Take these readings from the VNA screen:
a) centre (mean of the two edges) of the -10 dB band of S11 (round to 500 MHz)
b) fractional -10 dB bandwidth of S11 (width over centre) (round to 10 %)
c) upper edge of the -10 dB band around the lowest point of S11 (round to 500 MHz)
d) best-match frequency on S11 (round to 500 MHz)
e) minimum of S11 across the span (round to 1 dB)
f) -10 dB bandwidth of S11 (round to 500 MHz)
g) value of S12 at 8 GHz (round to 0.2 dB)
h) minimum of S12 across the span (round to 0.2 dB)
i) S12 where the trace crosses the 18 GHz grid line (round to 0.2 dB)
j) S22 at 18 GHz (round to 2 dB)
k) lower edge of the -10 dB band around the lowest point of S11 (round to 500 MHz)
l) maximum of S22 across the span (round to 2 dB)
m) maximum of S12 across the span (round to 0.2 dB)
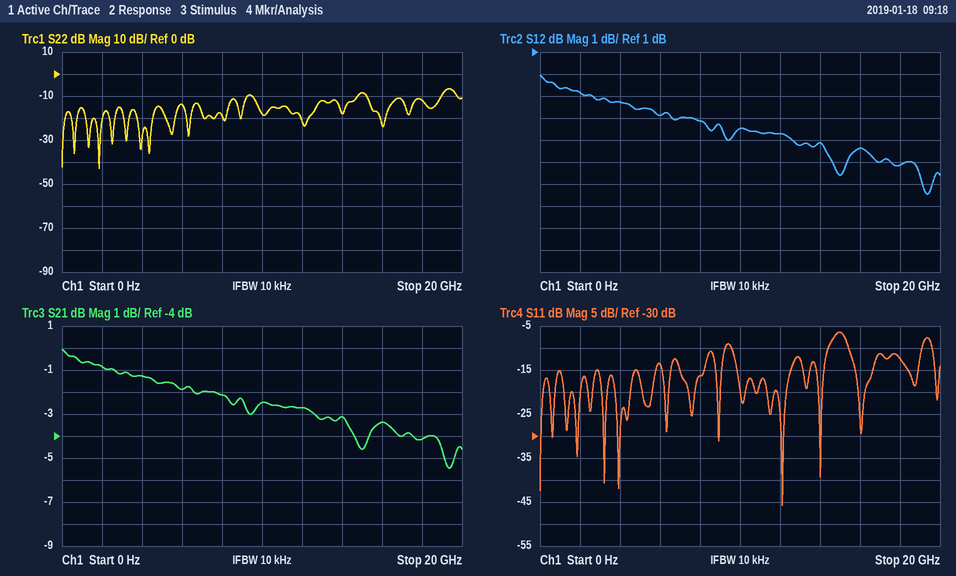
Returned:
12.0 GHz
40 %
14.5 GHz
12.0 GHz
-46 dB
5.0 GHz
-2.2 dB
-5.4 dB
-4.2 dB
-12 dB
9.5 GHz
-6 dB
0.0 dB
